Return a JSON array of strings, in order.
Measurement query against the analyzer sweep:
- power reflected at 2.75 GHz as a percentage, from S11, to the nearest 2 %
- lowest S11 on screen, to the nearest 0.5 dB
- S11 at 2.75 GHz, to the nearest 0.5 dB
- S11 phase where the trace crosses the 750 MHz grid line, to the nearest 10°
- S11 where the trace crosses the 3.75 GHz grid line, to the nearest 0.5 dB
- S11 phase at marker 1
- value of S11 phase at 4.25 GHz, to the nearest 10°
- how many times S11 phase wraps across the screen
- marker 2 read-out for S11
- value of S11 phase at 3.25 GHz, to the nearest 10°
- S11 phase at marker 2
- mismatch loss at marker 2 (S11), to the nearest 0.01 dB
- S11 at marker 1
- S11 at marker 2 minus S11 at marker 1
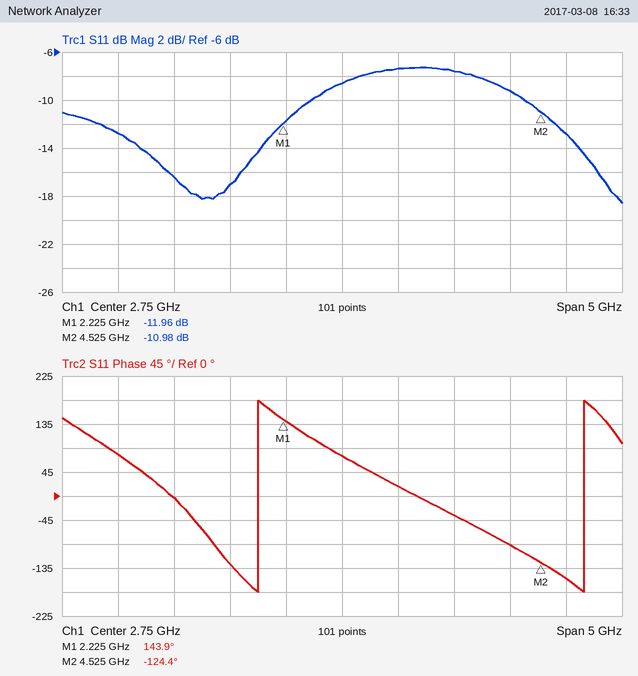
["14 %", "-18.5 dB", "-8.5 dB", "80°", "-7.5 dB", "143.9°", "-90°", "2", "-10.98 dB", "20°", "-124.4°", "0.36 dB", "-11.96 dB", "0.98 dB"]
